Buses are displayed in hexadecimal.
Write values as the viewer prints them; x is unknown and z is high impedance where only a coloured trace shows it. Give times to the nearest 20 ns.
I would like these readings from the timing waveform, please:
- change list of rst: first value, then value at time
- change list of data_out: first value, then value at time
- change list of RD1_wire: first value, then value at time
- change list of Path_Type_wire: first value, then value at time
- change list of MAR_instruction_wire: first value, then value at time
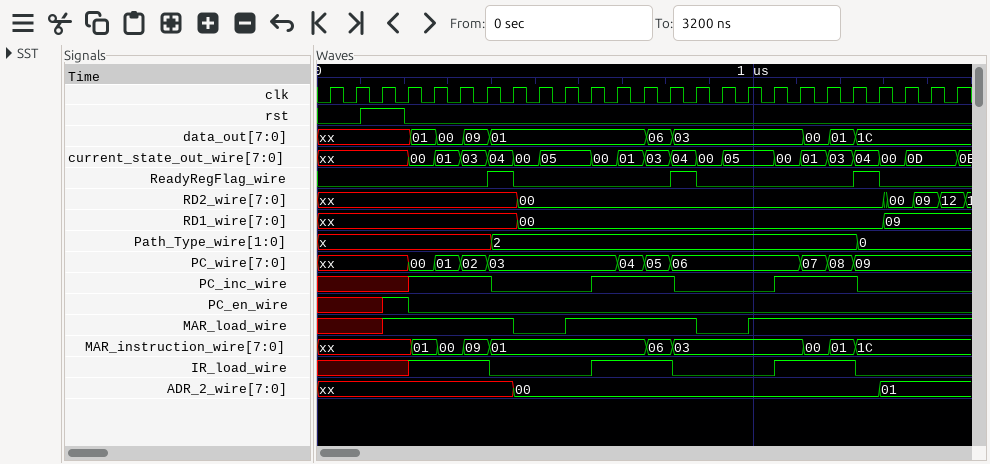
0, 1 at 100 ns, 0 at 200 ns
xx, 01 at 220 ns, 00 at 280 ns, 09 at 340 ns, 01 at 400 ns, 06 at 760 ns, 03 at 820 ns, 00 at 1120 ns, 01 at 1180 ns, 1C at 1240 ns
xx, 00 at 460 ns, 09 at 1300 ns
x, 2 at 400 ns, 0 at 1240 ns
xx, 01 at 220 ns, 00 at 280 ns, 09 at 340 ns, 01 at 400 ns, 06 at 760 ns, 03 at 820 ns, 00 at 1120 ns, 01 at 1180 ns, 1C at 1240 ns
